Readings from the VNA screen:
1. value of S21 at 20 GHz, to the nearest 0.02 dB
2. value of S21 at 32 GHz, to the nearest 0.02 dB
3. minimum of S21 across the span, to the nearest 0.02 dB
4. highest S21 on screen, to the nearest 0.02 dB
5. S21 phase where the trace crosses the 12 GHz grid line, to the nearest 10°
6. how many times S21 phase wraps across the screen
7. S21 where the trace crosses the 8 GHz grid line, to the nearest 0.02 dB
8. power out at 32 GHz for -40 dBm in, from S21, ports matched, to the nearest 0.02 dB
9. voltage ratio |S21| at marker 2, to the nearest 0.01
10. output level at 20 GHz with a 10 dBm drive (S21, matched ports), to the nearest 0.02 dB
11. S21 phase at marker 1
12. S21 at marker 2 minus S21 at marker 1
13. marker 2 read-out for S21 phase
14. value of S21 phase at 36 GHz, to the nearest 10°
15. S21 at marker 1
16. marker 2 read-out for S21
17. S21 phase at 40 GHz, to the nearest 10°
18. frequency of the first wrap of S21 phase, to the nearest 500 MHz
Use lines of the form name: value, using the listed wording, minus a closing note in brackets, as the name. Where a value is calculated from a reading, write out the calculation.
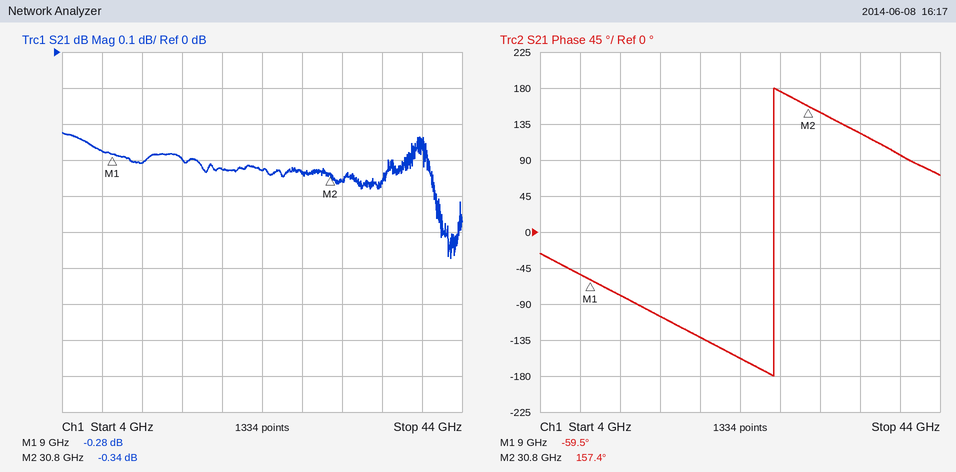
value of S21 at 20 GHz, to the nearest 0.02 dB: -0.32 dB
value of S21 at 32 GHz, to the nearest 0.02 dB: -0.36 dB
minimum of S21 across the span, to the nearest 0.02 dB: -0.58 dB
highest S21 on screen, to the nearest 0.02 dB: -0.22 dB
S21 phase where the trace crosses the 12 GHz grid line, to the nearest 10°: -80°
how many times S21 phase wraps across the screen: 1
S21 where the trace crosses the 8 GHz grid line, to the nearest 0.02 dB: -0.28 dB
power out at 32 GHz for -40 dBm in, from S21, ports matched, to the nearest 0.02 dB: -40 dBm + (-0.36 dB) = -40.36 dBm
voltage ratio |S21| at marker 2, to the nearest 0.01: 10^(-0.34/20) ≈ 0.96
output level at 20 GHz with a 10 dBm drive (S21, matched ports), to the nearest 0.02 dB: 10 dBm + (-0.32 dB) = 9.68 dBm
S21 phase at marker 1: -59.5°
S21 at marker 2 minus S21 at marker 1: -0.34 − (-0.28) = -0.06 dB
marker 2 read-out for S21 phase: 157.4°
value of S21 phase at 36 GHz, to the nearest 10°: 120°
S21 at marker 1: -0.28 dB
marker 2 read-out for S21: -0.34 dB
S21 phase at 40 GHz, to the nearest 10°: 100°
frequency of the first wrap of S21 phase, to the nearest 500 MHz: 27.5 GHz
